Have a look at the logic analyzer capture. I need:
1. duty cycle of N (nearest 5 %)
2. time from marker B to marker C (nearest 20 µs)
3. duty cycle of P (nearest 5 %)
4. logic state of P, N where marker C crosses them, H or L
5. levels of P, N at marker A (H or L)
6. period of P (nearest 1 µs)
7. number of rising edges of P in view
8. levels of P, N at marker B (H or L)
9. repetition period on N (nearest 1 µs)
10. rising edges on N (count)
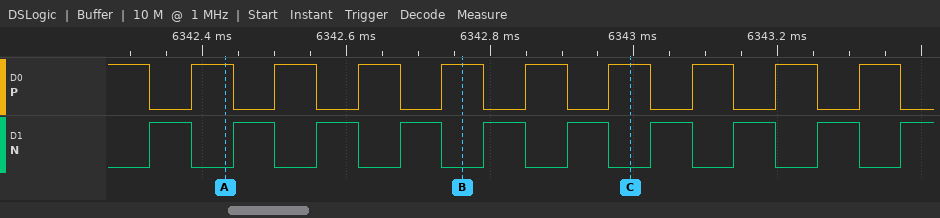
50 %
240 µs
50 %
P=H, N=L
P=H, N=L
116 µs
9
P=H, N=L
116 µs
10
